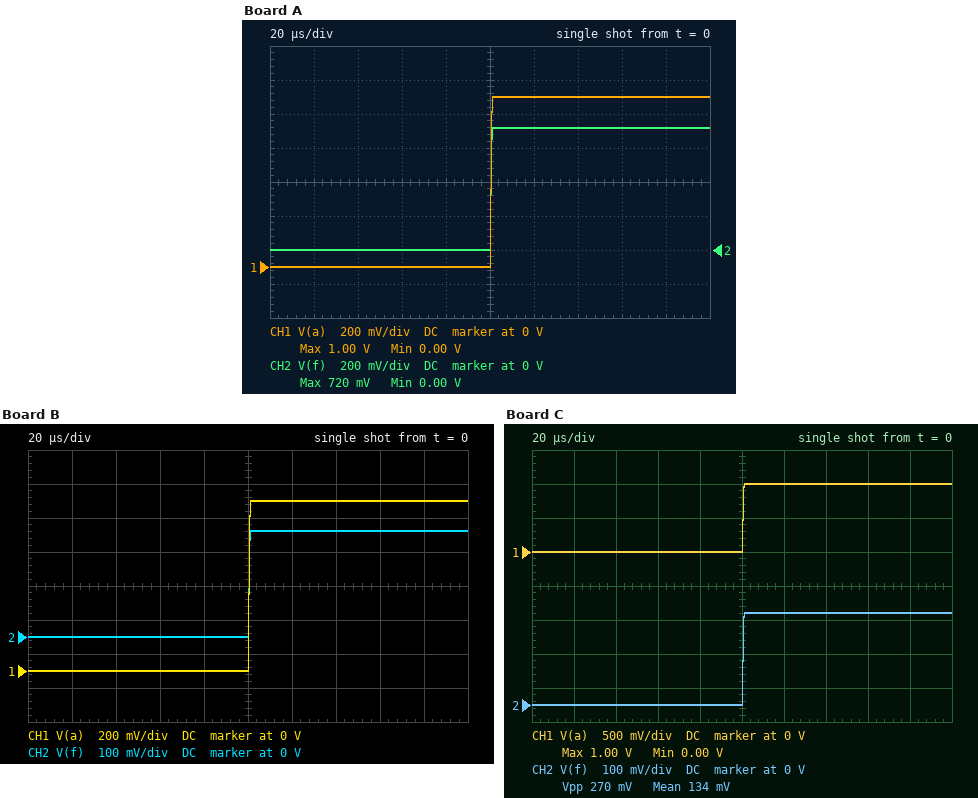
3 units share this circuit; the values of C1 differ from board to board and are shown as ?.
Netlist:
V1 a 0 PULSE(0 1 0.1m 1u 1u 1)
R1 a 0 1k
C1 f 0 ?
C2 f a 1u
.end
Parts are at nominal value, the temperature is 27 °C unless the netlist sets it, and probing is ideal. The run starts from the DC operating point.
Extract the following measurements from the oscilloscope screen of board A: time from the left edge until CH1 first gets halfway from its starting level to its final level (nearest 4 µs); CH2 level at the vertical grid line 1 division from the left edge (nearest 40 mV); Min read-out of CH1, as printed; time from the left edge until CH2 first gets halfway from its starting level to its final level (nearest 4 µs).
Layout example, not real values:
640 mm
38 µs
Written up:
100 µs
0 V
0.00 V
100 µs
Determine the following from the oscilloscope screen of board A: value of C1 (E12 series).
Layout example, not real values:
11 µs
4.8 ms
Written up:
390 nF
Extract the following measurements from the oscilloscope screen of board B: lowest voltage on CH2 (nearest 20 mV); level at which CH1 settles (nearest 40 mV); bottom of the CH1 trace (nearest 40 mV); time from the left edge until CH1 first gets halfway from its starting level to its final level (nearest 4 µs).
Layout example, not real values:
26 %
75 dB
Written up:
0 V
1.00 V
0 V
100 µs
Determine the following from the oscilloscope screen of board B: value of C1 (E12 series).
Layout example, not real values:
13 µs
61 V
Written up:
2.2 µF
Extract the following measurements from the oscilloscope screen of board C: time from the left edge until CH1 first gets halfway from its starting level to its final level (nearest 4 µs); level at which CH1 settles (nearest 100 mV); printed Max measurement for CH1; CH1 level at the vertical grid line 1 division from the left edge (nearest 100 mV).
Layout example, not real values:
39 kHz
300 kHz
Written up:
100 µs
1.0 V
1.00 V
0 V
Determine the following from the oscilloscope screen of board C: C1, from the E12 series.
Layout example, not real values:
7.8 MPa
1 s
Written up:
2.7 µF
